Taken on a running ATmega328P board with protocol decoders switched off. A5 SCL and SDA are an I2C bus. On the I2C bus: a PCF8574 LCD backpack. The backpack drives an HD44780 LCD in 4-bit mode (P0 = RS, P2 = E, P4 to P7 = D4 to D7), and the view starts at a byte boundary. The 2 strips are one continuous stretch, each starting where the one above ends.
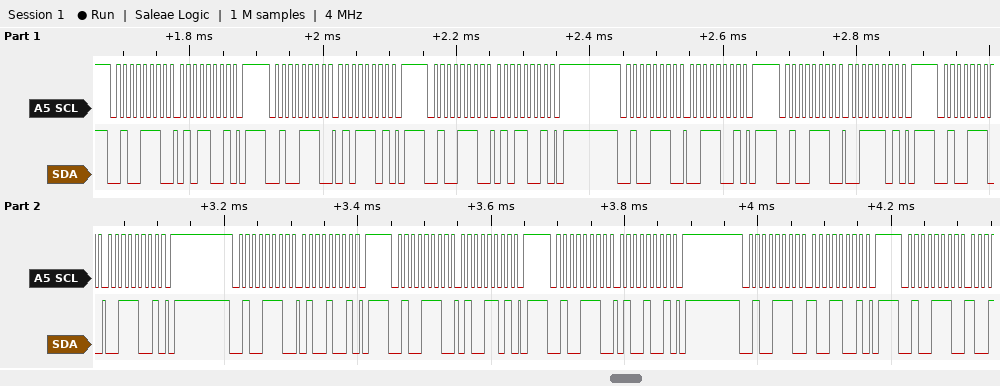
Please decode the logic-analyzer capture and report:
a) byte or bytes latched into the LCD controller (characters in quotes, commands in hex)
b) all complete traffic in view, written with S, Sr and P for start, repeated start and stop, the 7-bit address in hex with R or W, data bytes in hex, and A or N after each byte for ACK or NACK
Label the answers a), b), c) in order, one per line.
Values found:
a) 'S'
b) S 27W A 59 A P S 27W A 5D A P S 27W A 59 A P S 27W A 39 A P S 27W A 3D A P S 27W A 39 A P S 27W A 49 A P S 27W A 4D A P S 27W A 49 A P S 27W A 99 A P S 27W A
